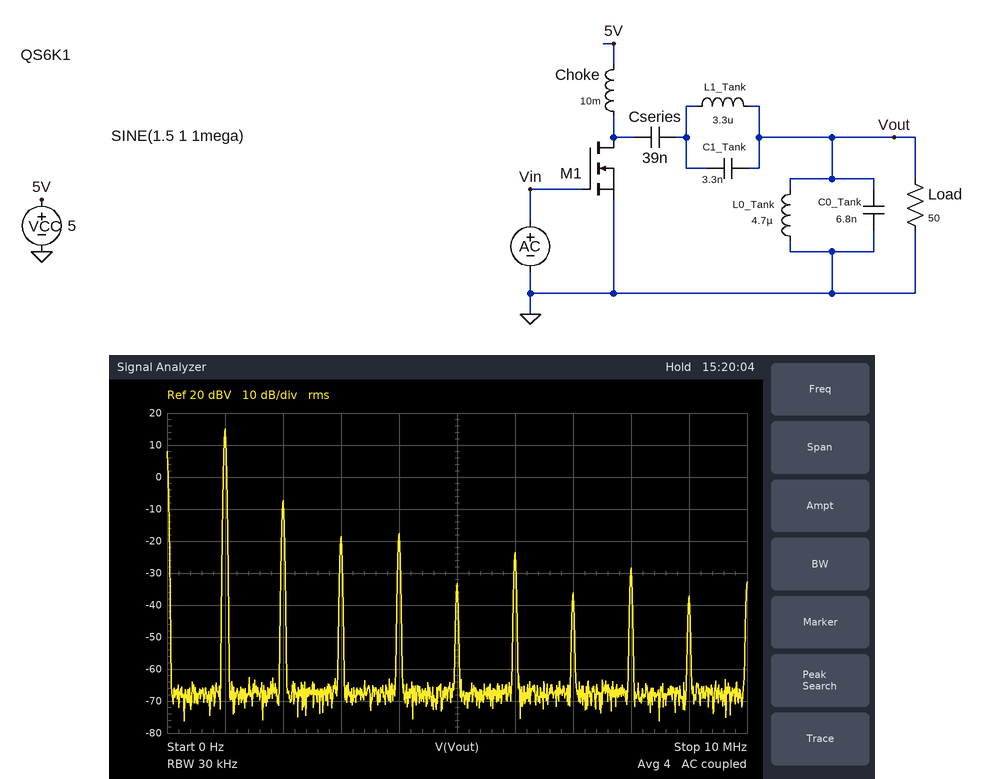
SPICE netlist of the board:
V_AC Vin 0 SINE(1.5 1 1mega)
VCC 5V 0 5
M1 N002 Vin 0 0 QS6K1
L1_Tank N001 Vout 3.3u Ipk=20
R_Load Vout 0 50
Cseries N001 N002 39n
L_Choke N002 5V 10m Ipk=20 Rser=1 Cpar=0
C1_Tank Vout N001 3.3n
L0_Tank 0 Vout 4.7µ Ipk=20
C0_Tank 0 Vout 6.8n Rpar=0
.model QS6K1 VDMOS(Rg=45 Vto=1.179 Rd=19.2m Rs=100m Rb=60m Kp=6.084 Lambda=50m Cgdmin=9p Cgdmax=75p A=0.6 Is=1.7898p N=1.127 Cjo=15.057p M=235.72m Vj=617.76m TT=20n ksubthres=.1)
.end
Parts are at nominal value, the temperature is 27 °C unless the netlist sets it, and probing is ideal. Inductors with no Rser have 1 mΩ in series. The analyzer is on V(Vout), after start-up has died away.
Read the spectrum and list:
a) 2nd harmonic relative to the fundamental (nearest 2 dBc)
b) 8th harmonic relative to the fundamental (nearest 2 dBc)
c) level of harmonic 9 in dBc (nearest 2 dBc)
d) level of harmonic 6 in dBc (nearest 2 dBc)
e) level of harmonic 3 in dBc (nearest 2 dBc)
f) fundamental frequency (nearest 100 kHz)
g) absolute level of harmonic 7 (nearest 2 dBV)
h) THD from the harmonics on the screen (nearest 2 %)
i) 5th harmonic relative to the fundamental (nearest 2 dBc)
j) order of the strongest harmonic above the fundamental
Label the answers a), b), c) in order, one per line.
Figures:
a) -22 dBc
b) -44 dBc
c) -52 dBc
d) -38 dBc
e) -34 dBc
f) 1.0 MHz
g) -36 dBV
h) 8 %
i) -48 dBc
j) 2
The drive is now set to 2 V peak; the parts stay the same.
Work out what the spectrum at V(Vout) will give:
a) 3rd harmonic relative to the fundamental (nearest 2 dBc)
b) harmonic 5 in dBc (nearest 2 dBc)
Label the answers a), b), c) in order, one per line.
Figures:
a) -30 dBc
b) -40 dBc
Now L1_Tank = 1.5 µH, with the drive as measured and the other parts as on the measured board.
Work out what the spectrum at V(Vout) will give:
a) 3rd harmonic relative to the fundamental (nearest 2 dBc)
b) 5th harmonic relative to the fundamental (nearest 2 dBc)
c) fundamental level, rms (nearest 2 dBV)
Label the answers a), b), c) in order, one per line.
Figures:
a) -30 dBc
b) -42 dBc
c) 16 dBV
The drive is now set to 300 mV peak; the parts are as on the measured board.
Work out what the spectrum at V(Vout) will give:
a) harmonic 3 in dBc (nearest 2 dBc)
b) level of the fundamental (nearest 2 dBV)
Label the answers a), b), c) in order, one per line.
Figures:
a) -40 dBc
b) 14 dBV
